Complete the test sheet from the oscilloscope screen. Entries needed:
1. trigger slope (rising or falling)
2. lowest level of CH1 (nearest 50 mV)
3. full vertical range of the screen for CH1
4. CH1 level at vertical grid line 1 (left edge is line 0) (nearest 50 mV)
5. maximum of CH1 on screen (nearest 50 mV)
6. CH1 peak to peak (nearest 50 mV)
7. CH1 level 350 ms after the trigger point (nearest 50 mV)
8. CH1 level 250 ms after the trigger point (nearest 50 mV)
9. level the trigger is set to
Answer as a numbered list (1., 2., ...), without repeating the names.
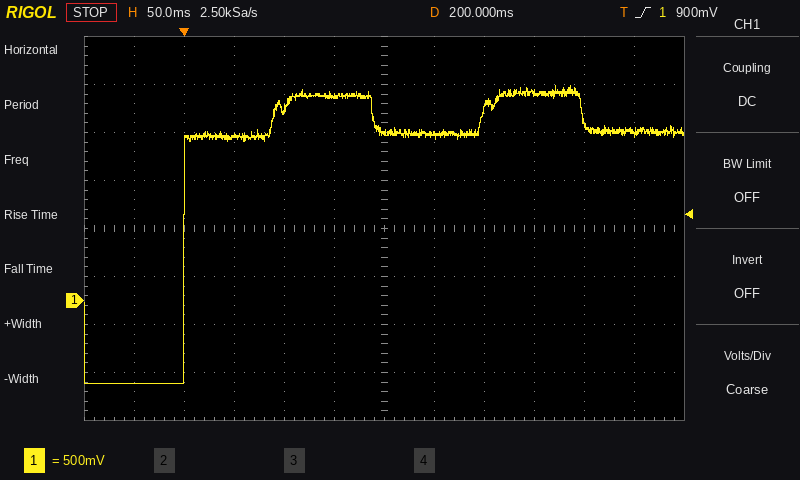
1. rising
2. -850 mV
3. 4 V
4. -850 mV
5. 2.25 V
6. 3.10 V
7. 2.15 V
8. 1.70 V
9. 900 mV
